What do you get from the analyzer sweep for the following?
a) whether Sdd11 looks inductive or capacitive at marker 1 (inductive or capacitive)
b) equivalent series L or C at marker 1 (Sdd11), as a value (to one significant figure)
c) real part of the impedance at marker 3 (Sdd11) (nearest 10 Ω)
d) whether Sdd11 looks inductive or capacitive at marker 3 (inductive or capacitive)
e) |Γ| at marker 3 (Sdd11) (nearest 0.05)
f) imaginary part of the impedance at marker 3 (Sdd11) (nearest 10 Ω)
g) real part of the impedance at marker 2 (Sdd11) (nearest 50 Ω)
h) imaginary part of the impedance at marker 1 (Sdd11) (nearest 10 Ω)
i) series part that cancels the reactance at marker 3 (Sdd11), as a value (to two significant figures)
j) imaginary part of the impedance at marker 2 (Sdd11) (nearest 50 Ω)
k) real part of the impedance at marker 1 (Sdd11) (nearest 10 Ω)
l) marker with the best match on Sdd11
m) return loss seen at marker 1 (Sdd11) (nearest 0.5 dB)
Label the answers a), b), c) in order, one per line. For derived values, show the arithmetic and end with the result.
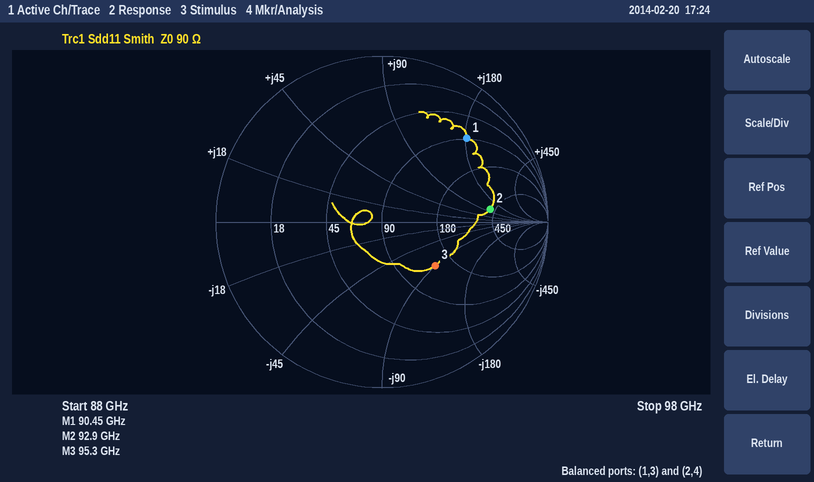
a) inductive
b) L = 180 Ω/(2π × 90.45 GHz) ≈ 317 pH, so 300 pH to one significant figure
c) 140 Ω
d) capacitive
e) 0.40
f) -90 Ω
g) 400 Ω
h) +180 Ω
i) L = 90 Ω/(2π × 95.3 GHz) ≈ 150 pH
j) +100 Ω
k) 90 Ω
l) marker 3
m) 3.0 dB
